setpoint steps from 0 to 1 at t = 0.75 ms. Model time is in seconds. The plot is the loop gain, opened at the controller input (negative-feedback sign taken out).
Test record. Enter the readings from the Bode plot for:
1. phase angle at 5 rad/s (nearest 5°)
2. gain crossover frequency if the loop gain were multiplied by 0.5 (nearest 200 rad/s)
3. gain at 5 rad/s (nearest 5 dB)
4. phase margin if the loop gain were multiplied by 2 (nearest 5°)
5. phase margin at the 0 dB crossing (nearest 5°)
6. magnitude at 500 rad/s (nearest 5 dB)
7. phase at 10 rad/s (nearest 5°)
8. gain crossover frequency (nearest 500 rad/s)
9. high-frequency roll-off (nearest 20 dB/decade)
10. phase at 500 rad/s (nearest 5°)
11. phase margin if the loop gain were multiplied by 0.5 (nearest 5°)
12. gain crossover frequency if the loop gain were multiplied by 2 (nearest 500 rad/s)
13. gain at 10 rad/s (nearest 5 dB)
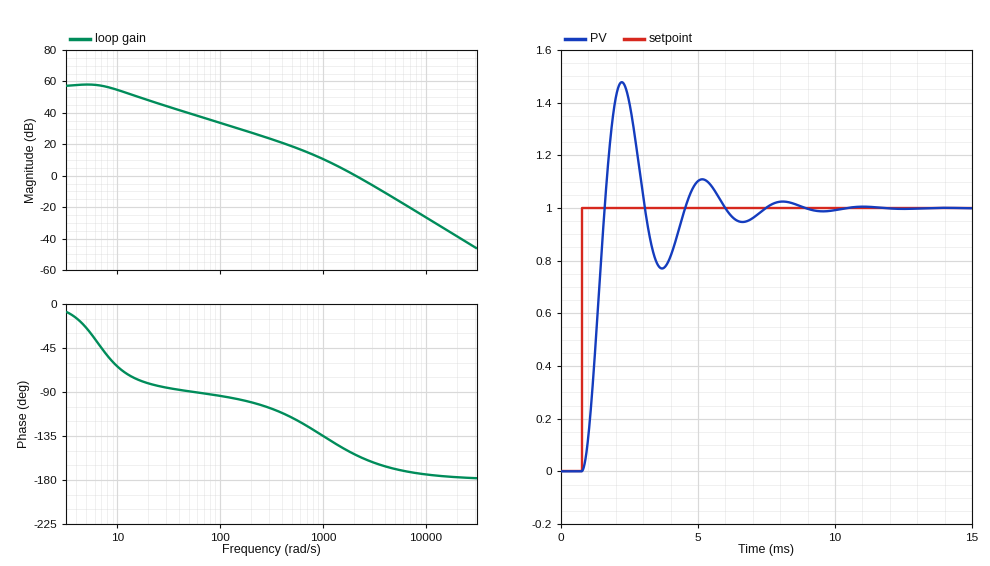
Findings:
-25°
1400 rad/s
60 dB
20°
25°
20 dB
-65°
2000 rad/s
-40 dB/decade
-115°
35°
3000 rad/s
55 dB
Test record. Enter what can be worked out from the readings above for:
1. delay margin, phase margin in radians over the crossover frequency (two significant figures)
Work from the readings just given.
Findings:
0.00022 s
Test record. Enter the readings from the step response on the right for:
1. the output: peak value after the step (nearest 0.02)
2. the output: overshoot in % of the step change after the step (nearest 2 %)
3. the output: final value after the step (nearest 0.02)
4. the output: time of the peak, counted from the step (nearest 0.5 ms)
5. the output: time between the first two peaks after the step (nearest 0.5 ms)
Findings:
1.48
48 %
1.00
1.5 ms
3.0 ms
